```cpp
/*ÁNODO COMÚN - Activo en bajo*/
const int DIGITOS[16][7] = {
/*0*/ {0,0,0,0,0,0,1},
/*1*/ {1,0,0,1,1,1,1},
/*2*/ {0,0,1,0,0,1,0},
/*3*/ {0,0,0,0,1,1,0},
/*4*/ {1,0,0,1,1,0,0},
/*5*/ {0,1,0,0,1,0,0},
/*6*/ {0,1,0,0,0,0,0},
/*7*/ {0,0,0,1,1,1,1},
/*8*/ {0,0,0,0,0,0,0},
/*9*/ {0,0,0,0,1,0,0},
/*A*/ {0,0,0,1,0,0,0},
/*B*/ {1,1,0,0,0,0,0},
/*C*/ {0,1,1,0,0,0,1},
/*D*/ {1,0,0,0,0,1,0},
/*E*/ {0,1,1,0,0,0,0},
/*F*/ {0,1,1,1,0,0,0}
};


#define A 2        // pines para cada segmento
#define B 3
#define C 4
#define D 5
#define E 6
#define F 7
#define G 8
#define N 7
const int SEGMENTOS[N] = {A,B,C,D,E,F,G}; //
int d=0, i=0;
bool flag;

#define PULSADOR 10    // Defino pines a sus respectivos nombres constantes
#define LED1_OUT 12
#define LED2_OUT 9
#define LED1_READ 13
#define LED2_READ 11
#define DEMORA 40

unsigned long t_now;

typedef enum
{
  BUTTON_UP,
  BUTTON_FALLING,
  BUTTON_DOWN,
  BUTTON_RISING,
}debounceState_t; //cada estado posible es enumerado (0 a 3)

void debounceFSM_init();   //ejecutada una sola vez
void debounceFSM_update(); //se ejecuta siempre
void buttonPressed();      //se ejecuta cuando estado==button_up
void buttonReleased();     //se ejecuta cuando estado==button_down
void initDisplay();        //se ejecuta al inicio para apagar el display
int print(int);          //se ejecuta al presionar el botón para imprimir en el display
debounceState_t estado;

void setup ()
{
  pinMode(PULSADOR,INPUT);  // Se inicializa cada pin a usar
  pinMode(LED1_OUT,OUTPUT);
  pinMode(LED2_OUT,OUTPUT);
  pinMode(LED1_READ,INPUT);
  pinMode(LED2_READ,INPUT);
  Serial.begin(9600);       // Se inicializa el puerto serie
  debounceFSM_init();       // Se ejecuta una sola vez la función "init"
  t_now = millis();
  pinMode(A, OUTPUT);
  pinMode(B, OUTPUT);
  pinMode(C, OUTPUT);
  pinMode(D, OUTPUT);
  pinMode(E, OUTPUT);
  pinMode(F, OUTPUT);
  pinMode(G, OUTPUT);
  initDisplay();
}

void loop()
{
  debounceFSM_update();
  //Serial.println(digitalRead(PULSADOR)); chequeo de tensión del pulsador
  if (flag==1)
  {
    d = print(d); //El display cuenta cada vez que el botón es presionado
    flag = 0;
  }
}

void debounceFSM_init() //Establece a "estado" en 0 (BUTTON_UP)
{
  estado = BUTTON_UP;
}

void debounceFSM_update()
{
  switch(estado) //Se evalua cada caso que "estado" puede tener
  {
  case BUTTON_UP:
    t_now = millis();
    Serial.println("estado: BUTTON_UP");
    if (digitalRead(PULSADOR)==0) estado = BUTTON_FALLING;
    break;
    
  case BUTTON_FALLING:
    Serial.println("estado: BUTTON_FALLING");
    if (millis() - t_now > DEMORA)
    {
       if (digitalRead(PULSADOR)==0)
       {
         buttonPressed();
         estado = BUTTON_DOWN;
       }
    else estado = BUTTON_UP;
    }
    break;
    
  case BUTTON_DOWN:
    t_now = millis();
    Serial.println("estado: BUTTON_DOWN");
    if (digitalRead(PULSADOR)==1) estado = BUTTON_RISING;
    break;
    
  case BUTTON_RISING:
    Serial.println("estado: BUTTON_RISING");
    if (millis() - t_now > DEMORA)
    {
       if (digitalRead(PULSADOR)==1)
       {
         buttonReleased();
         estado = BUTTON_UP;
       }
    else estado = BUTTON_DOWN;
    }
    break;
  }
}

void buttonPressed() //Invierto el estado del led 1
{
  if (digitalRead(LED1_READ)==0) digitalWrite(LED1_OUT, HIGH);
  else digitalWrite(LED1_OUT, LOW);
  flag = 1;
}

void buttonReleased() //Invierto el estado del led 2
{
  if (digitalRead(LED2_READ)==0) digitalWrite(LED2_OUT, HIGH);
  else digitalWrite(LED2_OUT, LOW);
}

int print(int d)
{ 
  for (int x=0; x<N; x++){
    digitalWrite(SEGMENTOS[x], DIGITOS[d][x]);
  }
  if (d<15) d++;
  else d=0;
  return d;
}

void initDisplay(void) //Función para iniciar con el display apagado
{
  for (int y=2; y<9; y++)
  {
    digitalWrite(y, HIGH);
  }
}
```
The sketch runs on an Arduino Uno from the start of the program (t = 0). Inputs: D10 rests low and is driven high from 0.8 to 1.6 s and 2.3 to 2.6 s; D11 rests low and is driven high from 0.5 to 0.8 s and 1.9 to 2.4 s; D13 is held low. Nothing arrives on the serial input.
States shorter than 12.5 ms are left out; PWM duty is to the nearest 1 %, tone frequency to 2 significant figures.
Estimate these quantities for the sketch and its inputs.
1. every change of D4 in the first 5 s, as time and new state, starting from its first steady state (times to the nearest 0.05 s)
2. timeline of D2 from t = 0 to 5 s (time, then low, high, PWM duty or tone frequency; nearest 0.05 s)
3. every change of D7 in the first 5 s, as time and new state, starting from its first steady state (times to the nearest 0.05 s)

0 s high; 0.05 s low; 2.65 s high
0 s high; 0.05 s low; 1.65 s high; 2.65 s low
0 s high; 0.05 s low; 1.65 s high
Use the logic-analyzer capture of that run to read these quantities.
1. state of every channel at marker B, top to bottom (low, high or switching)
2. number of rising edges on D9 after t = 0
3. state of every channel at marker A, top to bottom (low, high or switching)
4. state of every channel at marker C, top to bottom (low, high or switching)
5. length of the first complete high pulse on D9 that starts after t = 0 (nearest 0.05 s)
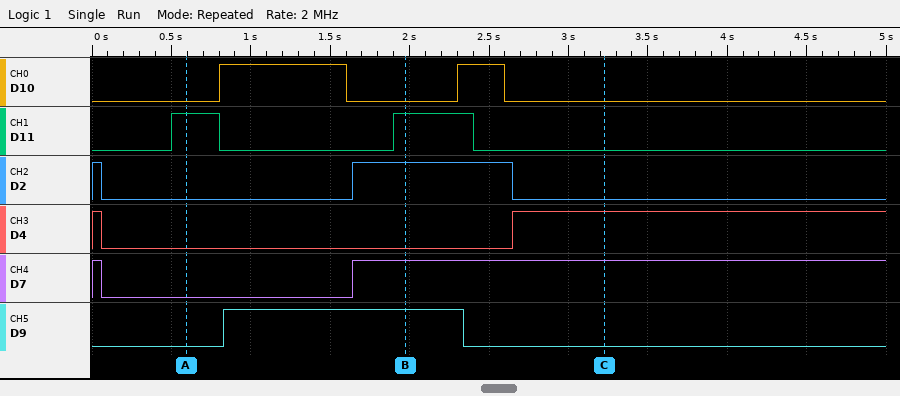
D10 low, D11 high, D2 high, D4 low, D7 high, D9 high
1
D10 low, D11 high, D2 low, D4 low, D7 low, D9 low
D10 low, D11 low, D2 low, D4 high, D7 high, D9 low
1.50 s
